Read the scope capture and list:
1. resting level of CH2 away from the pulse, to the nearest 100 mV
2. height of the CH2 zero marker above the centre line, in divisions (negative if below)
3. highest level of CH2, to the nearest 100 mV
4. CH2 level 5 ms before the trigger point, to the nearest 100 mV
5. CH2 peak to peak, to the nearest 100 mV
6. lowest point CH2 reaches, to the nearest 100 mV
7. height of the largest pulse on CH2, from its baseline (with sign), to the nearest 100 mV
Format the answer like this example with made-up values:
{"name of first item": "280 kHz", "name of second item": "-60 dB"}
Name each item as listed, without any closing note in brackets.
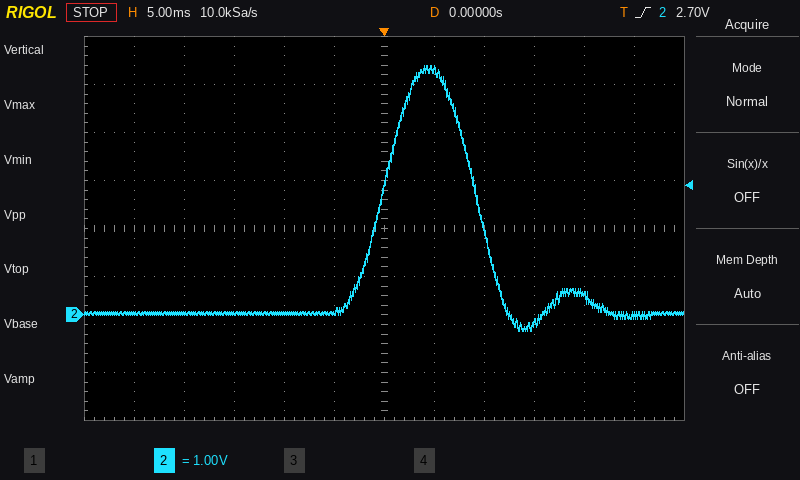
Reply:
{"resting level of CH2 away from the pulse, to the nearest 100 mV": "0.0 V", "height of the CH2 zero marker above the centre line, in divisions": "-1.8 div", "highest level of CH2, to the nearest 100 mV": "5.2 V", "CH2 level 5 ms before the trigger point, to the nearest 100 mV": "100 mV", "CH2 peak to peak, to the nearest 100 mV": "5.5 V", "lowest point CH2 reaches, to the nearest 100 mV": "-300 mV", "height of the largest pulse on CH2, from its baseline (with sign), to the nearest 100 mV": "+5.2 V"}
